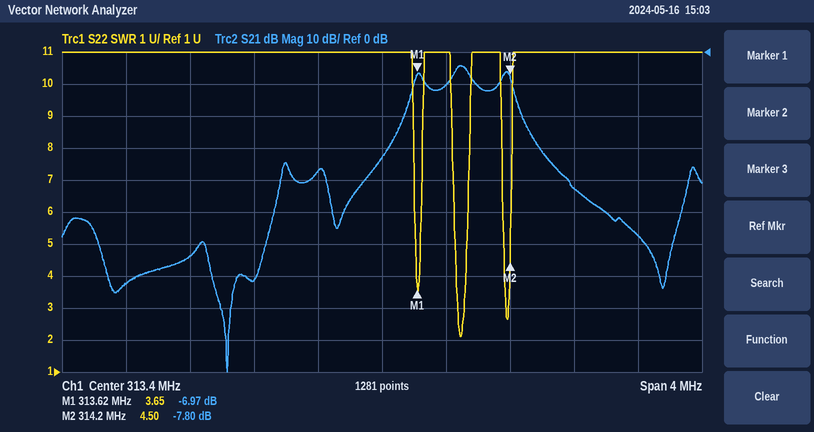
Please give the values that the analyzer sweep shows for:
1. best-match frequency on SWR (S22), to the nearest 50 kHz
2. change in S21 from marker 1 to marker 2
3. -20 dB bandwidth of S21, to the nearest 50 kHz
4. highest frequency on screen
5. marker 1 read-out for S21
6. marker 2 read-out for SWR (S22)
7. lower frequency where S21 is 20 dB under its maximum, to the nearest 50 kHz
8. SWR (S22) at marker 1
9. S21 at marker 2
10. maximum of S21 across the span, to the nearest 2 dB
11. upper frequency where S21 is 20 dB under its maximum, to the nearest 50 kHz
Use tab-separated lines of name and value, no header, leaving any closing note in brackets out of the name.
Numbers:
best-match frequency on SWR (S22), to the nearest 50 kHz	313.90 MHz
change in S21 from marker 1 to marker 2	-0.83 dB
-20 dB bandwidth of S21, to the nearest 50 kHz	800 kHz
highest frequency on screen	315.4 MHz
marker 1 read-out for S21	-6.97 dB
marker 2 read-out for SWR	4.50
lower frequency where S21 is 20 dB under its maximum, to the nearest 50 kHz	313.50 MHz
SWR (S22) at marker 1	3.65
S21 at marker 2	-7.80 dB
maximum of S21 across the span, to the nearest 2 dB	-4 dB
upper frequency where S21 is 20 dB under its maximum, to the nearest 50 kHz	314.30 MHz
